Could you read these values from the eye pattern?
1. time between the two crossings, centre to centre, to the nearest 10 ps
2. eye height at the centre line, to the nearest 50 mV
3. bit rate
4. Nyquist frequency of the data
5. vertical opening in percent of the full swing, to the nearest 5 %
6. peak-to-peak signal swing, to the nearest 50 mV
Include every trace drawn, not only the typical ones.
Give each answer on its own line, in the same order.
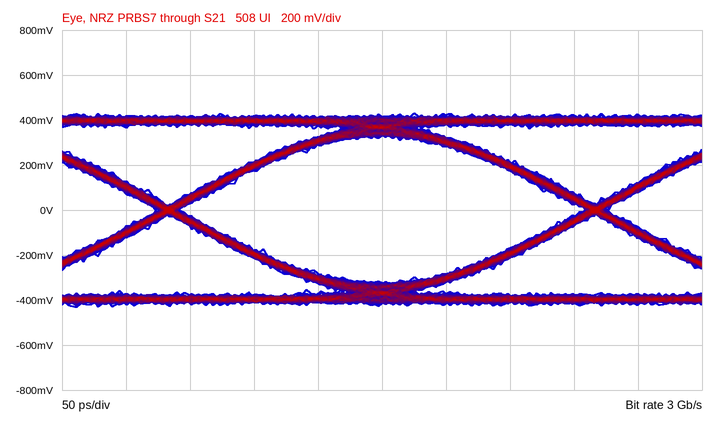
330 ps
650 mV
3 Gb/s
1.5 GHz
75 %
850 mV
